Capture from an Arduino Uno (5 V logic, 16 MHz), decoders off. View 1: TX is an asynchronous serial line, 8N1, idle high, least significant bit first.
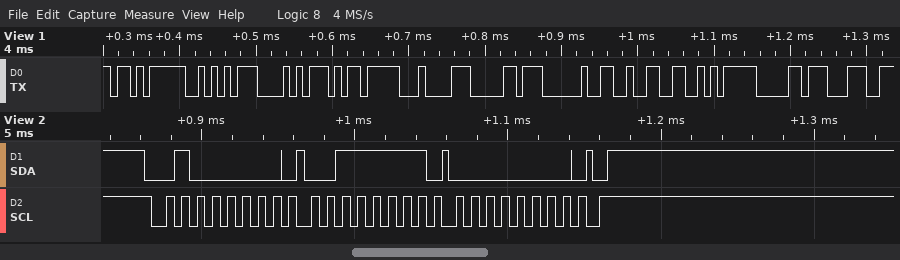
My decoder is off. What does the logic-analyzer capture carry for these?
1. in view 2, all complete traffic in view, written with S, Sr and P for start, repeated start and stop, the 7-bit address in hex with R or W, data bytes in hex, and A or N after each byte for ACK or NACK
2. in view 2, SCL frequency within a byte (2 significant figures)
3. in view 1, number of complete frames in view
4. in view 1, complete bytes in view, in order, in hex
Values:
S 20W A 3F A 00 A P
100 kHz
11
EB AA A8 ED 84 B0 20 32 EA B0 9C
